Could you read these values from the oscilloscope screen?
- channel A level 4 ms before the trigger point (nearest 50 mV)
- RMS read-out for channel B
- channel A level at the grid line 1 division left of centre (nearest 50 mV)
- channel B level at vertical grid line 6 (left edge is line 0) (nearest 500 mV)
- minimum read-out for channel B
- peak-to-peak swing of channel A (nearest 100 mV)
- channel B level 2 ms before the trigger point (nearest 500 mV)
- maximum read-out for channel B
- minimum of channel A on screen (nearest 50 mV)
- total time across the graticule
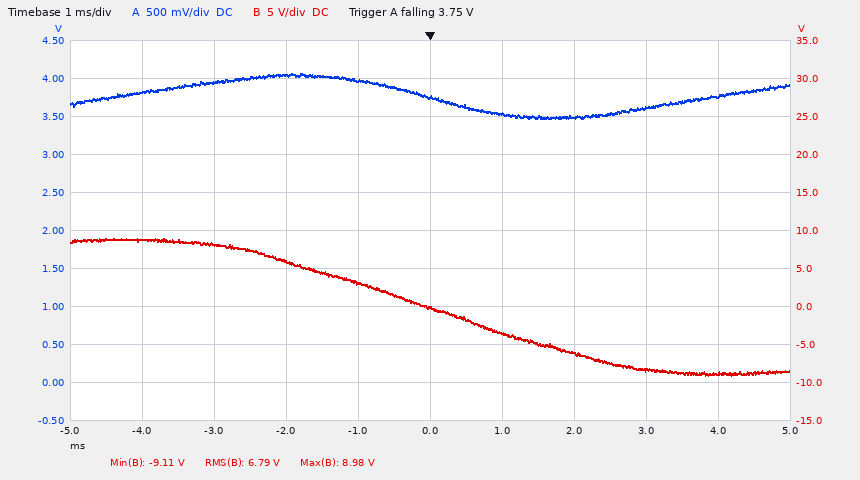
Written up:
3.80 V
6.79 V
3.95 V
-3.5 V
-9.11 V
600 mV
6.0 V
8.98 V
3.45 V
10 ms
